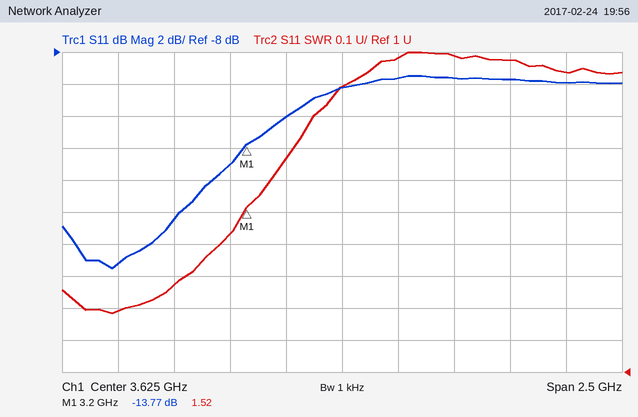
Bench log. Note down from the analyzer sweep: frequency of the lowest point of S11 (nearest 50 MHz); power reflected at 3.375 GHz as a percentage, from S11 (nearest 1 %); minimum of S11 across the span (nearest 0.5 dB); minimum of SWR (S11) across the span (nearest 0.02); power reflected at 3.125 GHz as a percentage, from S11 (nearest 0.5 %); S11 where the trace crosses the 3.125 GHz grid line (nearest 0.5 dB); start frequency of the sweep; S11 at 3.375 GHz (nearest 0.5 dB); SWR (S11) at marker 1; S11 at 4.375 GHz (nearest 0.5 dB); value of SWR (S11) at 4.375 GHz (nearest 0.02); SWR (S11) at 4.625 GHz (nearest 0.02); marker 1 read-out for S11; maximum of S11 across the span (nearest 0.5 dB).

2.60 GHz
6 %
-21.5 dB
1.18
3.0 %
-15.0 dB
2.375 GHz
-12.0 dB
1.52
-9.5 dB
1.98
1.94
-13.77 dB
-9.5 dB
